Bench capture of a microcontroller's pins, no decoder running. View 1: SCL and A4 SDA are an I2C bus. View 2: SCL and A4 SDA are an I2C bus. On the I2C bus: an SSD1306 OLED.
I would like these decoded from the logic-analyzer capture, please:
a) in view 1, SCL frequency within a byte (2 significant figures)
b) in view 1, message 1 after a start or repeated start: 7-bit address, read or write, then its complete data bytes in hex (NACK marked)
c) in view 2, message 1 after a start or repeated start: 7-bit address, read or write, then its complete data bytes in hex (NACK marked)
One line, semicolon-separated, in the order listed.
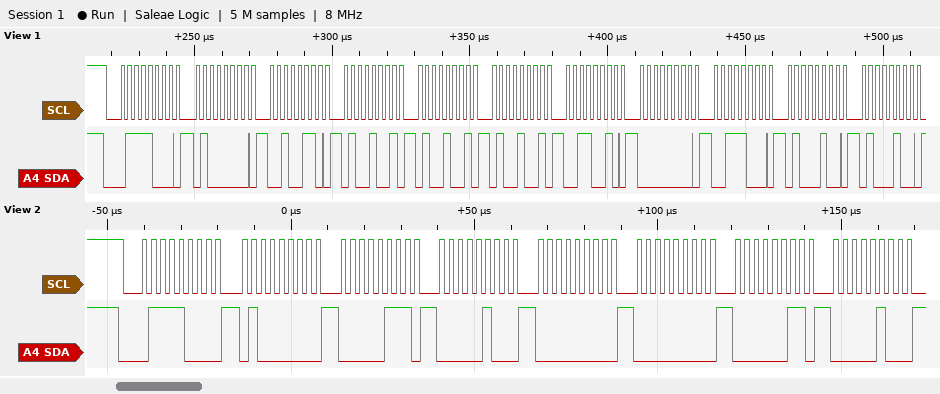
400 kHz; 0x3C write: 40 26 49 49 49 32 00 38 44 44; 0x3C write: 40 07 04 00 00 03 04
